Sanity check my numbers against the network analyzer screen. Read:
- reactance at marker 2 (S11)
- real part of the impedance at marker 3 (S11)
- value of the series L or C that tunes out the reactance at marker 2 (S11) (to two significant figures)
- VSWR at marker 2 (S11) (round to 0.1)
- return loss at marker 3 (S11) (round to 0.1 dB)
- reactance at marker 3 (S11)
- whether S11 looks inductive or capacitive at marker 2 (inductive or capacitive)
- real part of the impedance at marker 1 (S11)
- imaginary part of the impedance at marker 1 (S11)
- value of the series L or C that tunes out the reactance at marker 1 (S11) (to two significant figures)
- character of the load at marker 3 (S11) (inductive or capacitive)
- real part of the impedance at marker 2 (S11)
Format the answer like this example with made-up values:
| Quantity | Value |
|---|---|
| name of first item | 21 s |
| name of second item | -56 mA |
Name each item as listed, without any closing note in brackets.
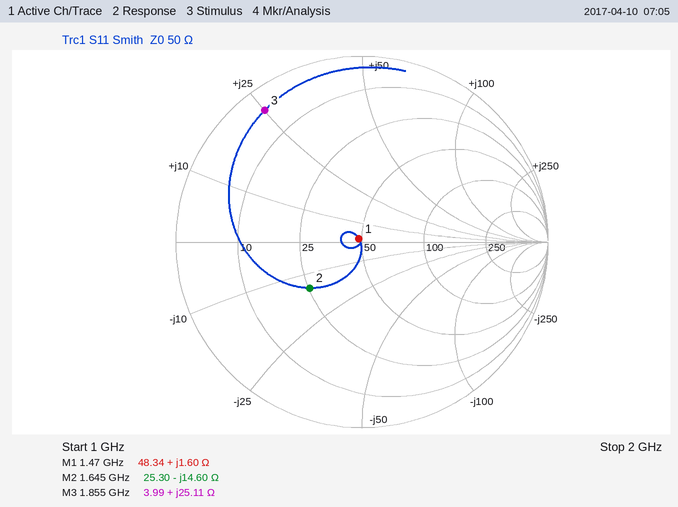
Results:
| Quantity | Value |
|---|---|
| reactance at marker 2 | -14.60 Ω |
| real part of the impedance at marker 3 | 3.99 Ω |
| value of the series L or C that tunes out the reactance at marker 2 (S11) | 1.4 nH |
| VSWR at marker 2 (S11) | 2.2 |
| return loss at marker 3 (S11) | 1.1 dB |
| reactance at marker 3 | +25.11 Ω |
| whether S11 looks inductive or capacitive at marker 2 | capacitive |
| real part of the impedance at marker 1 | 48.34 Ω |
| imaginary part of the impedance at marker 1 | +1.60 Ω |
| value of the series L or C that tunes out the reactance at marker 1 (S11) | 68 pF |
| character of the load at marker 3 (S11) | inductive |
| real part of the impedance at marker 2 | 25.30 Ω |
